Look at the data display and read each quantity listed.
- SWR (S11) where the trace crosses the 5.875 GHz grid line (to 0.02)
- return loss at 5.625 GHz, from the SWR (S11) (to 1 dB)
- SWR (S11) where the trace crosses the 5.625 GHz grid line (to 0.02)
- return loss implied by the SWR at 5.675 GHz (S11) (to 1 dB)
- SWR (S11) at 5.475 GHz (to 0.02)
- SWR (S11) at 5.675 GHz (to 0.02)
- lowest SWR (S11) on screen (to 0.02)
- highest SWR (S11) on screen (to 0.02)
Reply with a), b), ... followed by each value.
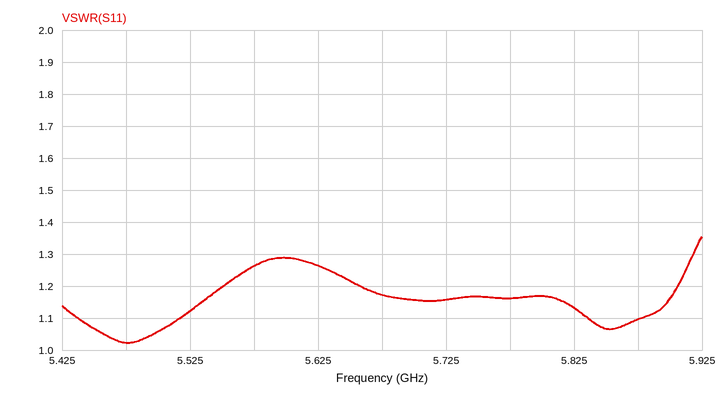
a) 1.10
b) 19 dB
c) 1.26
d) 22 dB
e) 1.02
f) 1.18
g) 1.02
h) 1.36
